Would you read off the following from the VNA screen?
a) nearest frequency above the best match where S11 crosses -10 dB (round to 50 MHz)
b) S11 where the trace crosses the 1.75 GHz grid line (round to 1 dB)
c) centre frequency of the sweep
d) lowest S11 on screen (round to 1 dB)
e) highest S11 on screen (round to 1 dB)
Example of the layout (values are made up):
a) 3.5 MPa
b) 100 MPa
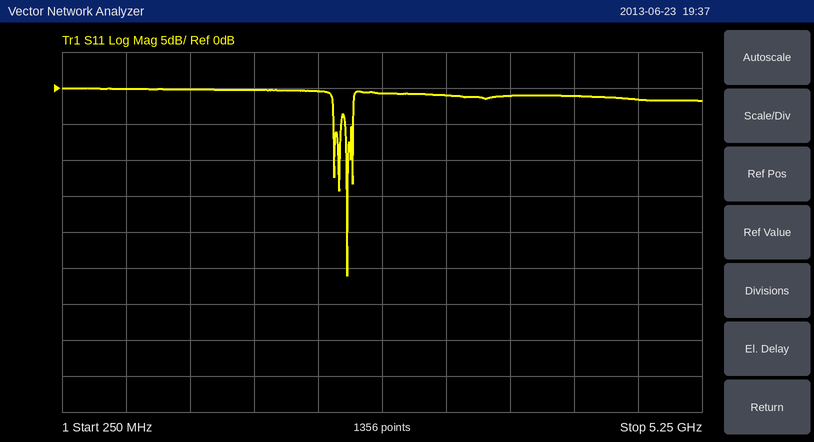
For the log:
a) 2.50 GHz
b) 0 dB
c) 2.75 GHz
d) -26 dB
e) 0 dB
